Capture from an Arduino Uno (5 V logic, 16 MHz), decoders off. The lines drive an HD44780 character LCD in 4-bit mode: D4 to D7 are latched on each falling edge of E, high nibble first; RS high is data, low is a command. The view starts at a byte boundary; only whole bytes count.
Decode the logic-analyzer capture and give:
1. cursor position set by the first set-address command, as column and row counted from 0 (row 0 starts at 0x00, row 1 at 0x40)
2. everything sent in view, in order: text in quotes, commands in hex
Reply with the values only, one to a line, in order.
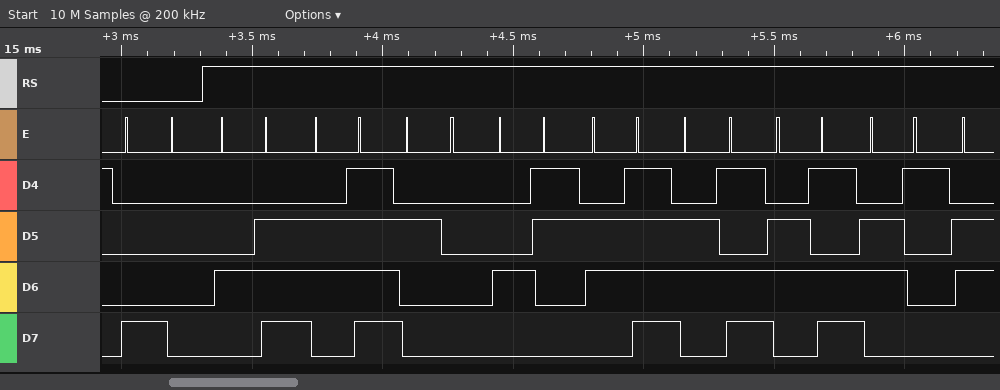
column 0, row 0
0x80 "No Comma"
